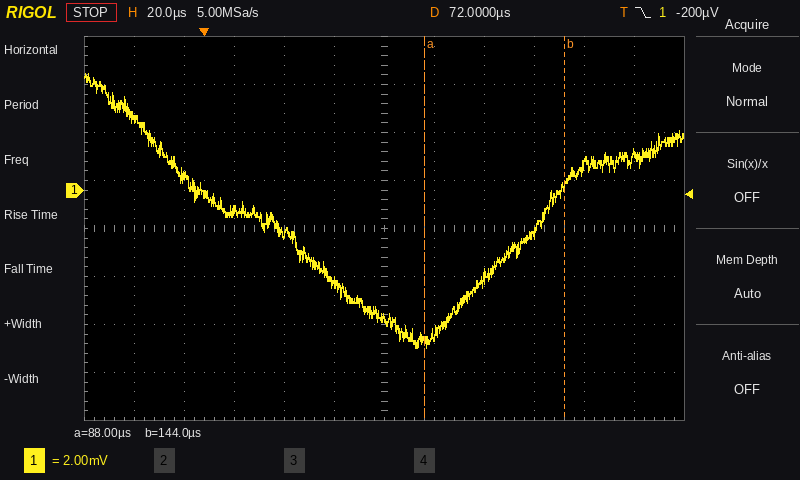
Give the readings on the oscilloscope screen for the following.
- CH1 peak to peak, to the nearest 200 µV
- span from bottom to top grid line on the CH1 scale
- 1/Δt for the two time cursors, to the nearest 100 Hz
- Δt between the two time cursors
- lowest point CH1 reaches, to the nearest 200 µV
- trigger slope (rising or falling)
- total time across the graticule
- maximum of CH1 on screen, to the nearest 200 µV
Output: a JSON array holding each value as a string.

["11.4 mV", "16 mV", "17.9 kHz", "56 µs", "-6.6 mV", "falling", "240 µs", "4.8 mV"]
